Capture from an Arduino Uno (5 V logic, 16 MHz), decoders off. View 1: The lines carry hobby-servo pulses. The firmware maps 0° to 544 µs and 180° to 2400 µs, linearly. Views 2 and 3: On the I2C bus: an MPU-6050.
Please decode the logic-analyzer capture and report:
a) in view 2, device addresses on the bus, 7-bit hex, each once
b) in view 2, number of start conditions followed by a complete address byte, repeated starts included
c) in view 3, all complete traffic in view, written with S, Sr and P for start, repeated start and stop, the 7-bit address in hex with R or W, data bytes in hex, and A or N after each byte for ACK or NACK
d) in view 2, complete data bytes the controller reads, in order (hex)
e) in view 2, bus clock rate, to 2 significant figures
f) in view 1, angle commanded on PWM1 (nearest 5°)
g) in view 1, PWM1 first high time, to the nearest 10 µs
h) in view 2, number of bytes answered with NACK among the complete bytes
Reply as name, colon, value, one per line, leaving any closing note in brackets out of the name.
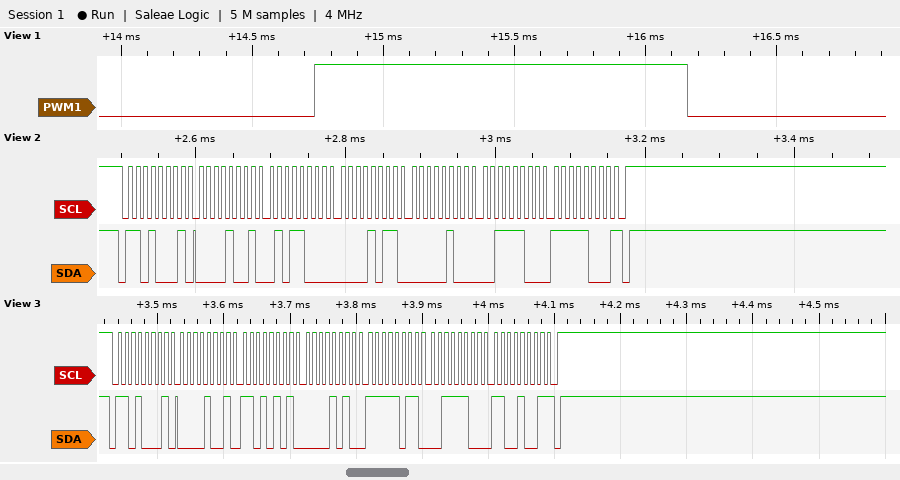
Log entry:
in view 2, device addresses on the bus, 7-bit hex, each once: 0x68
in view 2, number of start conditions followed by a complete address byte, repeated starts included: 1
in view 3, all complete traffic in view, written with S, Sr and P for start, repeated start and stop, the 7-bit address in hex with R or W, data bytes in hex, and A or N after each byte for ACK or NACK: S 68R A 09 A D5 A 0A A FB A 3C A C9 N P
in view 2, complete data bytes the controller reads, in order: 09 58 0B 04 3C F8
in view 2, bus clock rate, to 2 significant figures: 100 kHz
in view 1, angle commanded on PWM1: 85°
in view 1, PWM1 first high time, to the nearest 10 µs: 1420 µs
in view 2, number of bytes answered with NACK among the complete bytes: 1
